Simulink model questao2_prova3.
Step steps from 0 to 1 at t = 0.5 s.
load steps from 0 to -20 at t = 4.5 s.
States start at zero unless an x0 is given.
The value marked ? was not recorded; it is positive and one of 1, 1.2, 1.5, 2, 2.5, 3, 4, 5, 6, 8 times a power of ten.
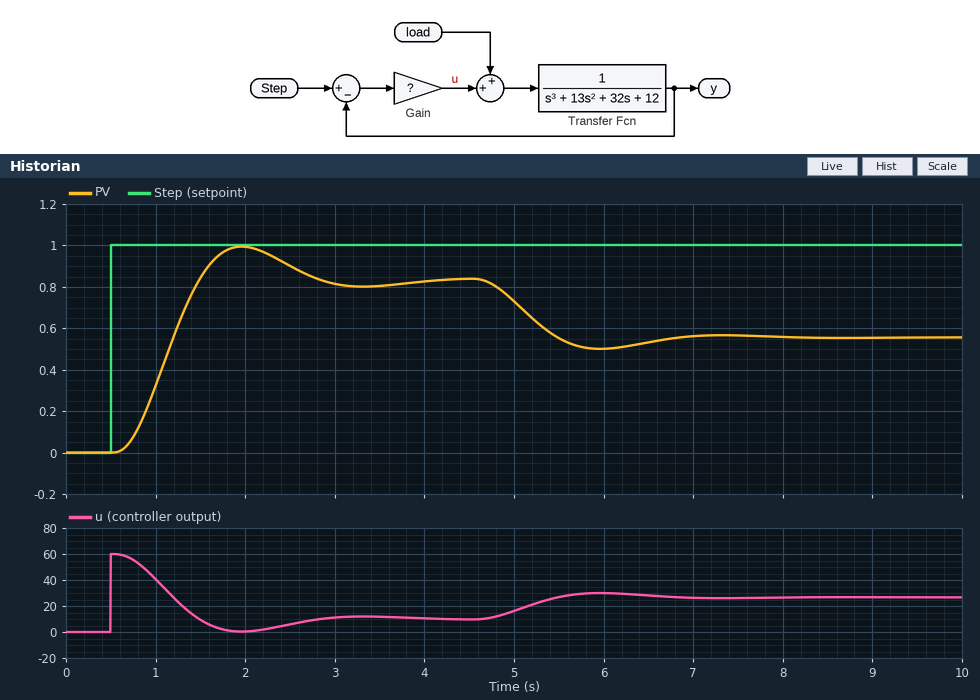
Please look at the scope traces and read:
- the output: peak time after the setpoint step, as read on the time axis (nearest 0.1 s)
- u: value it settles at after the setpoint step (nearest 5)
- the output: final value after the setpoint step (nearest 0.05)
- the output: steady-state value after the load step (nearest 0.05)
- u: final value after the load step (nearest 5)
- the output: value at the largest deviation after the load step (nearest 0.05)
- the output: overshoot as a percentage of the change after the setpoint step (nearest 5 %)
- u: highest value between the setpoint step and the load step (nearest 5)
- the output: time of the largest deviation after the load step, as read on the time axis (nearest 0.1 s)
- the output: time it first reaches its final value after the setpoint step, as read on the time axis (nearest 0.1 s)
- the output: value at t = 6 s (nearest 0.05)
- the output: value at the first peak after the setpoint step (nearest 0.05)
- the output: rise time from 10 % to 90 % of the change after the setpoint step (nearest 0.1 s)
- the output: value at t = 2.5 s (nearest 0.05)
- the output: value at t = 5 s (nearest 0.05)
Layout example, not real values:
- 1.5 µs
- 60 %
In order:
- 2.0 s
- 10
- 0.85
- 0.55
- 25
- 0.50
- 20 %
- 60
- 6.0 s
- 1.5 s
- 0.50
- 1.00
- 0.6 s
- 0.90
- 0.75
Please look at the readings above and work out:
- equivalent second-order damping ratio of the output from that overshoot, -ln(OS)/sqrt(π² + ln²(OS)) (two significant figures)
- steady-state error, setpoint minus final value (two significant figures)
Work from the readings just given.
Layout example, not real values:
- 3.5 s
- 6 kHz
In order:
- 0.46
- 0.15
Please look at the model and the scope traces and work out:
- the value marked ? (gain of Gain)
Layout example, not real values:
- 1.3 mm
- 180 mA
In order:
- 60
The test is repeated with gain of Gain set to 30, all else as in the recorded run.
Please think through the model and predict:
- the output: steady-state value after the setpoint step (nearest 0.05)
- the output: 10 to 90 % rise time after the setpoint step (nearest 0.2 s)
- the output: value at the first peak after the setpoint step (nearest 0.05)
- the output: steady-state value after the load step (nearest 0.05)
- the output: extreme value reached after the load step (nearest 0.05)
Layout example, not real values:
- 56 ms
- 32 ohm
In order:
- 0.70
- 1.0 s
- 0.75
- 0.25
- 0.20
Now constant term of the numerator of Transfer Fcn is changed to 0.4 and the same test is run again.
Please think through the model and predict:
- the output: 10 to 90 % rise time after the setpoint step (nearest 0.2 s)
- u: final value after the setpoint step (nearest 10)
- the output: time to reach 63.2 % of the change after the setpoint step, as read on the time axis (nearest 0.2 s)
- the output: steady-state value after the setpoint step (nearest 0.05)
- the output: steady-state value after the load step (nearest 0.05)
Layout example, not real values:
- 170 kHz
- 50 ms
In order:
- 1.2 s
- 20
- 1.6 s
- 0.65
- 0.45
